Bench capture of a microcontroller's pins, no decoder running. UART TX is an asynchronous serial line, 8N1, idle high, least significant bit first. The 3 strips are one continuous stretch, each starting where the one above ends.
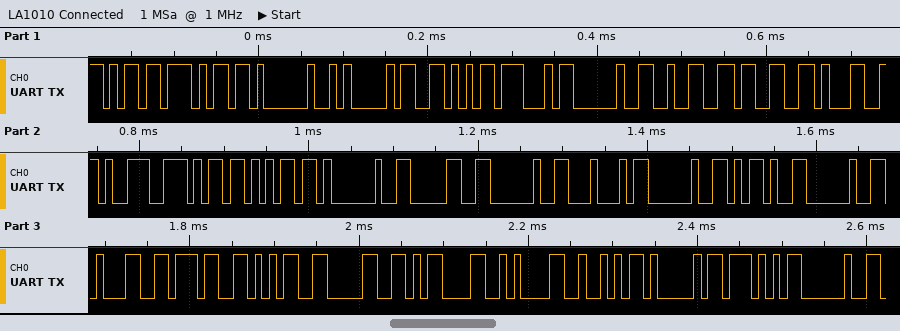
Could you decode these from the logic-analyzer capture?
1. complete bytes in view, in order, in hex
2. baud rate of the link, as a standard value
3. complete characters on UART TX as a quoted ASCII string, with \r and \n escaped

0x6D 0x6D 0x20 0x41 0x56 0x47 0x20 0x32 0x33 0x31 0x39 0x6D 0x6D 0x20 0x30 0x20 0x44 0x20 0x2D 0x20 0x31 0x37 0x35 0x30 0x0D 0x0A 0x52 0x41 0x57 0x20
115200 baud
"mm AVG 2319mm 0 D - 1750\r\nRAW "
